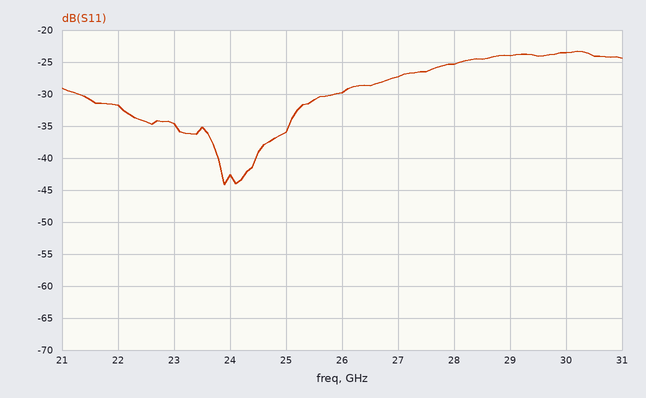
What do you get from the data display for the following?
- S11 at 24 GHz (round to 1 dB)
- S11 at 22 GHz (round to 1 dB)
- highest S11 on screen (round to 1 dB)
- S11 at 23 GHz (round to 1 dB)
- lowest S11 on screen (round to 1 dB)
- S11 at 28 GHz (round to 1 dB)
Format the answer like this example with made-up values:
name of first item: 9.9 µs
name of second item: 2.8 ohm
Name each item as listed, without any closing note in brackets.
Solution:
S11 at 24 GHz: -43 dB
S11 at 22 GHz: -32 dB
highest S11 on screen: -23 dB
S11 at 23 GHz: -35 dB
lowest S11 on screen: -44 dB
S11 at 28 GHz: -25 dB
